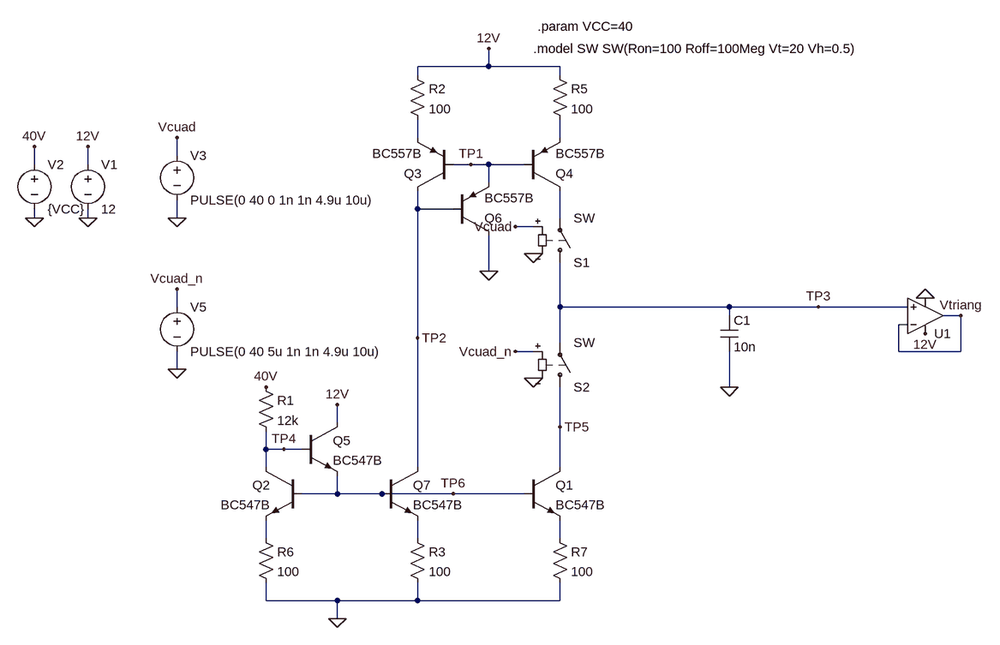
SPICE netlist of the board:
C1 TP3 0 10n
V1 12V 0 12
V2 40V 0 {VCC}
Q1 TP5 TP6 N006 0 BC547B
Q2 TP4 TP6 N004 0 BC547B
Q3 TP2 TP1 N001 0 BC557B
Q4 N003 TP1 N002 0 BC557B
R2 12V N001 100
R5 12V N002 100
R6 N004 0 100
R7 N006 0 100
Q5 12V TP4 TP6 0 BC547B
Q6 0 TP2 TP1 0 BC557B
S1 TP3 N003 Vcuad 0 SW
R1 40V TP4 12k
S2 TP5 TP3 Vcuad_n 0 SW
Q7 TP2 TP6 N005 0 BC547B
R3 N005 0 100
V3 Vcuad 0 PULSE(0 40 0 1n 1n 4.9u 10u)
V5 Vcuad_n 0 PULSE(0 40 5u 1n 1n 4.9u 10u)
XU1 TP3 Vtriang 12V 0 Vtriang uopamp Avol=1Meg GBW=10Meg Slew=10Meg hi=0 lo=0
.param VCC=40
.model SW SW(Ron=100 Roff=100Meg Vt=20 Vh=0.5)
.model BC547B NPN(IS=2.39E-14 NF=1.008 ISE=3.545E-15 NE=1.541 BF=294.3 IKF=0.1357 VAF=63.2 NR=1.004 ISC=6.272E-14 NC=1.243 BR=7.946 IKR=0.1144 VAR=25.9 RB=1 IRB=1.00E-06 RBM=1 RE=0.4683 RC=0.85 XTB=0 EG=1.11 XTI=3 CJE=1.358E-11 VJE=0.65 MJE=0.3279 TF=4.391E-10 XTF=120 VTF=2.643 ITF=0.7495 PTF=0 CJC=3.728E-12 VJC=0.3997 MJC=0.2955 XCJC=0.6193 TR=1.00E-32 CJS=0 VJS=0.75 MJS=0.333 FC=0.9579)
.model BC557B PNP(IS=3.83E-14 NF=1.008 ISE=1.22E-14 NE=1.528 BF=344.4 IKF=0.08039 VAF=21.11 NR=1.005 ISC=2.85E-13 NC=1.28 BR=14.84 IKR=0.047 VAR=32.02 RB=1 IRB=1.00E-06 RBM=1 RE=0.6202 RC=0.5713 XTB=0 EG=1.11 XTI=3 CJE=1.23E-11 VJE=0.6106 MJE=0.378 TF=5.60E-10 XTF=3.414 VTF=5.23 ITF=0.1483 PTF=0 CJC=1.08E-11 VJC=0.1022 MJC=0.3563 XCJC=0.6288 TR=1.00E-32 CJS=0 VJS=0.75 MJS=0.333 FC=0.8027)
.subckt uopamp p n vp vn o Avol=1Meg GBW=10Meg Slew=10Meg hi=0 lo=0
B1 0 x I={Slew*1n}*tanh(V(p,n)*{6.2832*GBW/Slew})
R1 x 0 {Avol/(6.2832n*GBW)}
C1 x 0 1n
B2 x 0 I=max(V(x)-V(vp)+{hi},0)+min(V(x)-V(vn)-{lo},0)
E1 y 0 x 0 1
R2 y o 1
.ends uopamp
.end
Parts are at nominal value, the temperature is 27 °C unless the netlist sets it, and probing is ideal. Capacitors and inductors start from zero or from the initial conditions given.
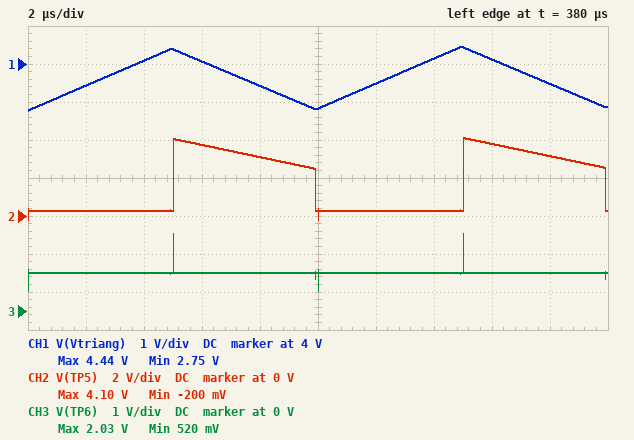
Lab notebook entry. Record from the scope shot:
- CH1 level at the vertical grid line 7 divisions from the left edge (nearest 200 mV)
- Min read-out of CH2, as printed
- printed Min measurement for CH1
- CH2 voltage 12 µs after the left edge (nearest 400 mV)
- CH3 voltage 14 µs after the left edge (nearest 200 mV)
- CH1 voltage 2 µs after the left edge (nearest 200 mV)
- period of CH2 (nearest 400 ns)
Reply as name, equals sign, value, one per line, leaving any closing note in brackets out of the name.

CH1 level at the vertical grid line 7 divisions from the left edge = 4.2 V
Min read-out of CH2, as printed = -200 mV
printed Min measurement for CH1 = 2.75 V
CH2 voltage 12 µs after the left edge = 400 mV
CH3 voltage 14 µs after the left edge = 1.0 V
CH1 voltage 2 µs after the left edge = 3.4 V
period of CH2 = 10.0 µs
